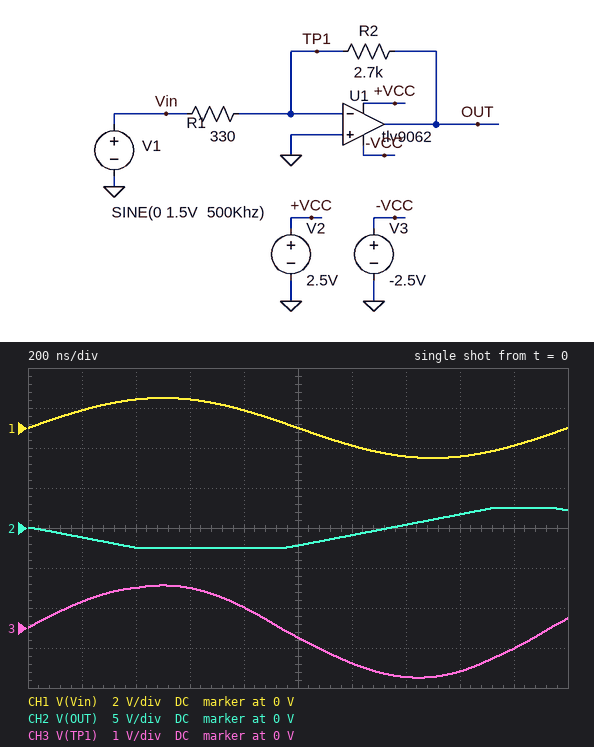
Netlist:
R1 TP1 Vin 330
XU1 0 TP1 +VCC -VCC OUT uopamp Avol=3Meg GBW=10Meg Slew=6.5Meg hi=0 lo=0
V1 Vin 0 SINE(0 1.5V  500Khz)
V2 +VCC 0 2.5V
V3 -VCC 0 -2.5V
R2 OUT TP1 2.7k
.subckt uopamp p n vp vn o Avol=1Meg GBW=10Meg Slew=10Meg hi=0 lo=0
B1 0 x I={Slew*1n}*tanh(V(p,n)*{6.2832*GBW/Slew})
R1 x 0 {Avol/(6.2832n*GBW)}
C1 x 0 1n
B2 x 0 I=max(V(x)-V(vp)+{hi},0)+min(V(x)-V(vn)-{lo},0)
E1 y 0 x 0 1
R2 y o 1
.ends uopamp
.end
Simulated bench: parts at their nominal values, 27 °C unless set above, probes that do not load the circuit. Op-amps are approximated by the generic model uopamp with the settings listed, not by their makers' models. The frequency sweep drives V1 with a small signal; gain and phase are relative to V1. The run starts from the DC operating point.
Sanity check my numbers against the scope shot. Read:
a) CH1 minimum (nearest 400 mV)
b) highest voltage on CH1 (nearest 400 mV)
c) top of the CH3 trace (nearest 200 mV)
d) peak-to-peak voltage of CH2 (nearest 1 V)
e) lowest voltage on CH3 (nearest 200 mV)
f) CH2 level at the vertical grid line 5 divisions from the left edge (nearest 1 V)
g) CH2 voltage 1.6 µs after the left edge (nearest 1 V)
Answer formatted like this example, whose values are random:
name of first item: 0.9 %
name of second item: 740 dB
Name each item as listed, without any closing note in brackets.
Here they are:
CH1 minimum: -1.6 V
highest voltage on CH1: 1.6 V
top of the CH3 trace: 1.0 V
peak-to-peak voltage of CH2: 5 V
lowest voltage on CH3: -1.2 V
CH2 level at the vertical grid line 5 divisions from the left edge: -2 V
CH2 voltage 1.6 µs after the left edge: 2 V
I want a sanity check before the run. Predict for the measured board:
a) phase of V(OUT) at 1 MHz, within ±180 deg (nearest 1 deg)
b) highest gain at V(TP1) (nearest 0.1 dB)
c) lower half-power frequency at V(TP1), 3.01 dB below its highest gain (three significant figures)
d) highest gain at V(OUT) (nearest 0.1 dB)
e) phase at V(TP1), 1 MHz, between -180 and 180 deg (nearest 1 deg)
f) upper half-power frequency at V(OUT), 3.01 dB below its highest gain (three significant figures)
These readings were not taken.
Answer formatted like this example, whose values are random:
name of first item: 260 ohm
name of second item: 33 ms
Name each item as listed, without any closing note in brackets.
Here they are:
phase of V(OUT) at 1 MHz, within ±180 deg: 137 deg
highest gain at V(TP1): -1.0 dB
lower half-power frequency at V(TP1), 3.01 dB below its highest gain: 1.09 MHz
highest gain at V(OUT): 18.3 dB
phase at V(TP1), 1 MHz, between -180 and 180 deg: 47 deg
upper half-power frequency at V(OUT), 3.01 dB below its highest gain: 1.09 MHz
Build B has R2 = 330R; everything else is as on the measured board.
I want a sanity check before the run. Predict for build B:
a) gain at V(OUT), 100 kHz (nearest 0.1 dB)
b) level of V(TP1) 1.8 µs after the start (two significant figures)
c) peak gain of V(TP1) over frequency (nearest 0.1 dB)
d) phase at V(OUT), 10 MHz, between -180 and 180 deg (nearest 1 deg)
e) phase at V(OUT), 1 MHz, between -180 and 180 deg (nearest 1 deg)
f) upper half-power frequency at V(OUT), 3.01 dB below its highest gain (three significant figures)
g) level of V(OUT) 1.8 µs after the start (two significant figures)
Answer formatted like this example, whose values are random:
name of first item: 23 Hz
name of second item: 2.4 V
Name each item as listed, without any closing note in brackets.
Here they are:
gain at V(OUT), 100 kHz: 0 dB
level of V(TP1) 1.8 µs after the start: 60 mV
peak gain of V(TP1) over frequency: -6.0 dB
phase at V(OUT), 10 MHz, between -180 and 180 deg: 116 deg
phase at V(OUT), 1 MHz, between -180 and 180 deg: 169 deg
upper half-power frequency at V(OUT), 3.01 dB below its highest gain: 4.99 MHz
level of V(OUT) 1.8 µs after the start: 1.0 V
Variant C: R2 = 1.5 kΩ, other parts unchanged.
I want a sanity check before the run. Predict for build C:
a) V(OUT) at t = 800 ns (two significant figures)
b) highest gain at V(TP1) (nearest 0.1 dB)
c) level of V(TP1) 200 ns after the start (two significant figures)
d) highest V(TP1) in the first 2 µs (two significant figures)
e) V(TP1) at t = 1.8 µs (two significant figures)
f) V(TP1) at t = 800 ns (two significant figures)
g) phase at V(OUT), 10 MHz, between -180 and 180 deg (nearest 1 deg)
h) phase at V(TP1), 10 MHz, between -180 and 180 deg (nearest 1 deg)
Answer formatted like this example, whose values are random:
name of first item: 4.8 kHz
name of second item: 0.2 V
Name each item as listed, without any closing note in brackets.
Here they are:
V(OUT) at t = 800 ns: -2.5 V
highest gain at V(TP1): -1.7 dB
level of V(TP1) 200 ns after the start: 510 mV
highest V(TP1) in the first 2 µs: 780 mV
V(TP1) at t = 1.8 µs: -270 mV
V(TP1) at t = 800 ns: 270 mV
phase at V(OUT), 10 MHz, between -180 and 180 deg: 100 deg
phase at V(TP1), 10 MHz, between -180 and 180 deg: 10 deg
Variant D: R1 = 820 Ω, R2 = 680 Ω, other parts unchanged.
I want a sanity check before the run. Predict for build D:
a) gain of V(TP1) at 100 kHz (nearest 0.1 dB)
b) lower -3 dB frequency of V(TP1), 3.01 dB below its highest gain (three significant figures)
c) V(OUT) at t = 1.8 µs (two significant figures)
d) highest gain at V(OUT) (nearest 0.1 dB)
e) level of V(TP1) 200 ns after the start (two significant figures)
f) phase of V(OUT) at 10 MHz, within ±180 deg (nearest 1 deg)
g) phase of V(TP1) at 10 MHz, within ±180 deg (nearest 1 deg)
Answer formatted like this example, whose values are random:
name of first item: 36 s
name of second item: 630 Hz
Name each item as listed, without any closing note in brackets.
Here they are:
gain of V(TP1) at 100 kHz: -41.6 dB
lower -3 dB frequency of V(TP1), 3.01 dB below its highest gain: 5.46 MHz
V(OUT) at t = 1.8 µs: 820 mV
highest gain at V(OUT): -1.6 dB
level of V(TP1) 200 ns after the start: 60 mV
phase of V(OUT) at 10 MHz, within ±180 deg: 119 deg
phase of V(TP1) at 10 MHz, within ±180 deg: 29 deg
